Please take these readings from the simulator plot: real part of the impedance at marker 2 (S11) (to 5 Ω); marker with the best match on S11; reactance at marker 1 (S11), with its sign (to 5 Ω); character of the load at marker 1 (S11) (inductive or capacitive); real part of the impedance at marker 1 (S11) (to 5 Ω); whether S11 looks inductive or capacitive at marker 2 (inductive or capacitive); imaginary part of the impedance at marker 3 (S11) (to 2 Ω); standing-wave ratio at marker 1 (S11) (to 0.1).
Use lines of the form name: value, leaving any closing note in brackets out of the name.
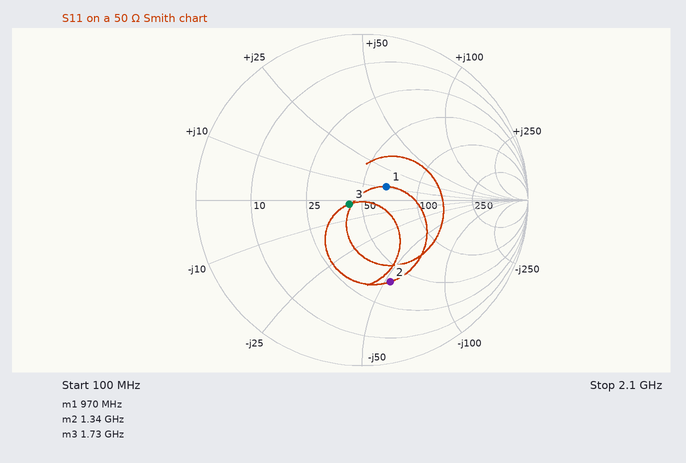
real part of the impedance at marker 2 (S11): 40 Ω
marker with the best match on S11: marker 3
reactance at marker 1 (S11), with its sign: +10 Ω
character of the load at marker 1 (S11): inductive
real part of the impedance at marker 1 (S11): 65 Ω
whether S11 looks inductive or capacitive at marker 2: capacitive
imaginary part of the impedance at marker 3 (S11): -2 Ω
standing-wave ratio at marker 1 (S11): 1.4
